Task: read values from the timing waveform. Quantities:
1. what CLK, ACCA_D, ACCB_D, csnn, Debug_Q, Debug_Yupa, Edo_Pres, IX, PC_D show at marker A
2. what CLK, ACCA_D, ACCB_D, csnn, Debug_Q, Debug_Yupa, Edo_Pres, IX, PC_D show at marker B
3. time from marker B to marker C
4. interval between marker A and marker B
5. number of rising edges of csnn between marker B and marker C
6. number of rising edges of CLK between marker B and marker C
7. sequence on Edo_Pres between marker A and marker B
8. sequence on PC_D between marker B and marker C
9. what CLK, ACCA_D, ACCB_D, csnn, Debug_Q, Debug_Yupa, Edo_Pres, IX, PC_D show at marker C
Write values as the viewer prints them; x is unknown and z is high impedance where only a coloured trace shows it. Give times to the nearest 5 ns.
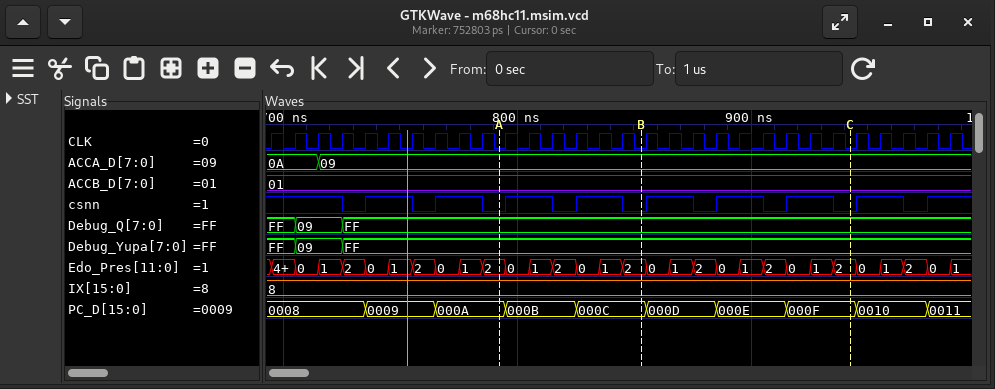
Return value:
CLK=0, ACCA_D=09, ACCB_D=01, csnn=0, Debug_Q=FF, Debug_Yupa=FF, Edo_Pres=2, IX=8, PC_D=000A
CLK=0, ACCA_D=09, ACCB_D=01, csnn=0, Debug_Q=FF, Debug_Yupa=FF, Edo_Pres=2, IX=8, PC_D=000C
90 ns
60 ns
3
9
2, 0, 1, 2, 0, 1, 2
000C, 000D, 000E, 000F
CLK=0, ACCA_D=09, ACCB_D=01, csnn=0, Debug_Q=FF, Debug_Yupa=FF, Edo_Pres=2, IX=8, PC_D=000F
